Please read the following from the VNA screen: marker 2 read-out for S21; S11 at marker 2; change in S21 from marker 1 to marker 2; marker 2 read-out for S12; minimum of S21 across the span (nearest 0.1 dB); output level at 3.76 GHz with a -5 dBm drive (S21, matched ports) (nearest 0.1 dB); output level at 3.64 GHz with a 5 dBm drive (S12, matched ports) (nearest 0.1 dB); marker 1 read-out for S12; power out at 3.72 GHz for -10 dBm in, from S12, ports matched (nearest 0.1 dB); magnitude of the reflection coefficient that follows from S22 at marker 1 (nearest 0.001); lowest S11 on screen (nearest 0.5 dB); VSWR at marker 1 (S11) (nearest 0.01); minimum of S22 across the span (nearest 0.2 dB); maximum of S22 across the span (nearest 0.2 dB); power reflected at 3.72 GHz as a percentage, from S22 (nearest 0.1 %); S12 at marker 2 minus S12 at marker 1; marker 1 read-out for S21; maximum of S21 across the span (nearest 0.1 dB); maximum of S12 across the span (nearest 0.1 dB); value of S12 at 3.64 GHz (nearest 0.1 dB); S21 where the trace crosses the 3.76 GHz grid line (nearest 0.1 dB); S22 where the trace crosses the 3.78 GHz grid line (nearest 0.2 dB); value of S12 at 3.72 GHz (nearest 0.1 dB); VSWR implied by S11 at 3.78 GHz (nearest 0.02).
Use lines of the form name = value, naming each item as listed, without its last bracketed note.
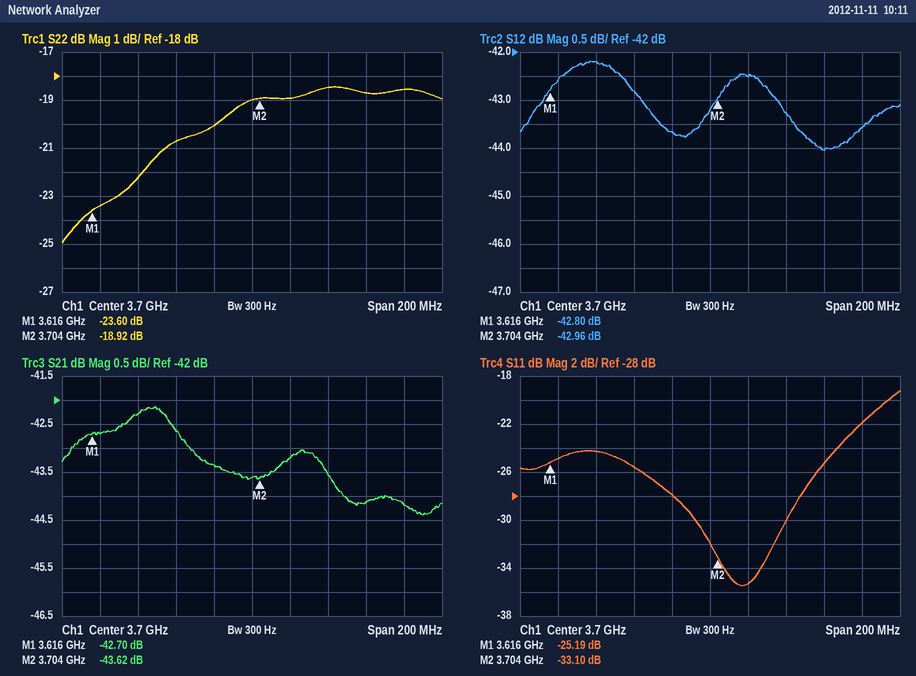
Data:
marker 2 read-out for S21 = -43.62 dB
S11 at marker 2 = -33.10 dB
change in S21 from marker 1 to marker 2 = -0.92 dB
marker 2 read-out for S12 = -42.96 dB
minimum of S21 across the span = -44.4 dB
output level at 3.76 GHz with a -5 dBm drive (S21, matched ports) = -49.1 dBm
output level at 3.64 GHz with a 5 dBm drive (S12, matched ports) = -37.2 dBm
marker 1 read-out for S12 = -42.80 dB
power out at 3.72 GHz for -10 dBm in, from S12, ports matched = -52.5 dBm
magnitude of the reflection coefficient that follows from S22 at marker 1 = 0.066
lowest S11 on screen = -35.5 dB
VSWR at marker 1 (S11) = 1.12
minimum of S22 across the span = -25.0 dB
maximum of S22 across the span = -18.4 dB
power reflected at 3.72 GHz as a percentage, from S22 = 1.3 %
S12 at marker 2 minus S12 at marker 1 = -0.16 dB
marker 1 read-out for S21 = -42.70 dB
maximum of S21 across the span = -42.1 dB
maximum of S12 across the span = -42.2 dB
value of S12 at 3.64 GHz = -42.2 dB
S21 where the trace crosses the 3.76 GHz grid line = -44.1 dB
S22 where the trace crosses the 3.78 GHz grid line = -18.6 dB
value of S12 at 3.72 GHz = -42.5 dB
VSWR implied by S11 at 3.78 GHz = 1.18
